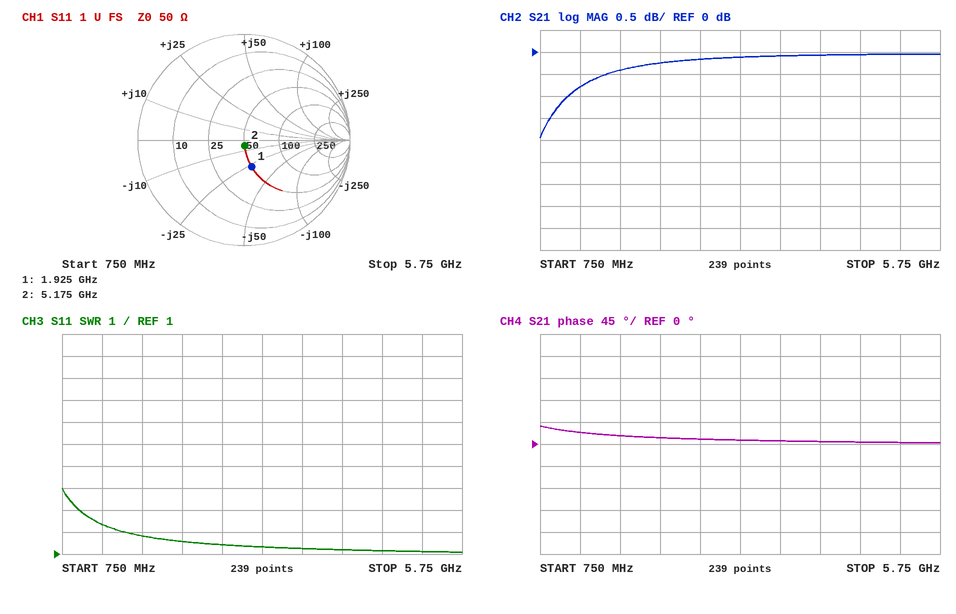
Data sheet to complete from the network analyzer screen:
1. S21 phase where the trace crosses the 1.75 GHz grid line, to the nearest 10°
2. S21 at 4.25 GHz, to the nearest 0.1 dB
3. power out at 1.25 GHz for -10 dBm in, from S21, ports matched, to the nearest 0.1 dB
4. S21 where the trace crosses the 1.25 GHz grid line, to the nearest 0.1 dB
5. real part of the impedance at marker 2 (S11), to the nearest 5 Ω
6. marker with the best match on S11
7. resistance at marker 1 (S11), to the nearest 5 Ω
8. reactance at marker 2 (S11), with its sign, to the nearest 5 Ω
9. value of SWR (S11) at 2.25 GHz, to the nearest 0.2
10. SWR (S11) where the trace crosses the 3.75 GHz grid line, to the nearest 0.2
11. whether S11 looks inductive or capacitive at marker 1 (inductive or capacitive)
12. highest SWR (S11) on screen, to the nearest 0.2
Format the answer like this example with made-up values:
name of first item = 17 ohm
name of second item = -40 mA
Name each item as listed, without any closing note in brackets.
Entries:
S21 phase where the trace crosses the 1.75 GHz grid line, to the nearest 10° = 20°
S21 at 4.25 GHz, to the nearest 0.1 dB = -0.1 dB
power out at 1.25 GHz for -10 dBm in, from S21, ports matched, to the nearest 0.1 dB = -10.8 dBm
S21 where the trace crosses the 1.25 GHz grid line, to the nearest 0.1 dB = -0.8 dB
real part of the impedance at marker 2 (S11), to the nearest 5 Ω = 50 Ω
marker with the best match on S11 = marker 2
resistance at marker 1 (S11), to the nearest 5 Ω = 50 Ω
reactance at marker 2 (S11), with its sign, to the nearest 5 Ω = -5 Ω
value of SWR (S11) at 2.25 GHz, to the nearest 0.2 = 1.6
SWR (S11) where the trace crosses the 3.75 GHz grid line, to the nearest 0.2 = 1.2
whether S11 looks inductive or capacitive at marker 1 = capacitive
highest SWR (S11) on screen, to the nearest 0.2 = 4.0
